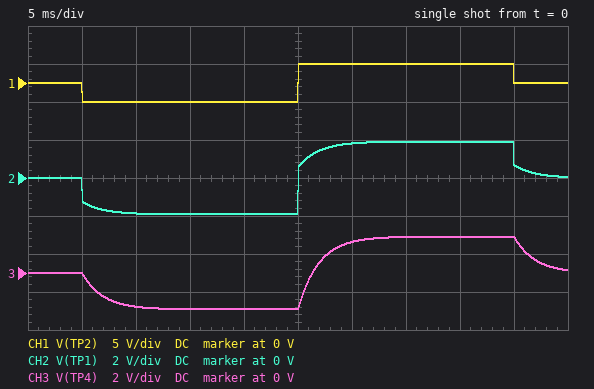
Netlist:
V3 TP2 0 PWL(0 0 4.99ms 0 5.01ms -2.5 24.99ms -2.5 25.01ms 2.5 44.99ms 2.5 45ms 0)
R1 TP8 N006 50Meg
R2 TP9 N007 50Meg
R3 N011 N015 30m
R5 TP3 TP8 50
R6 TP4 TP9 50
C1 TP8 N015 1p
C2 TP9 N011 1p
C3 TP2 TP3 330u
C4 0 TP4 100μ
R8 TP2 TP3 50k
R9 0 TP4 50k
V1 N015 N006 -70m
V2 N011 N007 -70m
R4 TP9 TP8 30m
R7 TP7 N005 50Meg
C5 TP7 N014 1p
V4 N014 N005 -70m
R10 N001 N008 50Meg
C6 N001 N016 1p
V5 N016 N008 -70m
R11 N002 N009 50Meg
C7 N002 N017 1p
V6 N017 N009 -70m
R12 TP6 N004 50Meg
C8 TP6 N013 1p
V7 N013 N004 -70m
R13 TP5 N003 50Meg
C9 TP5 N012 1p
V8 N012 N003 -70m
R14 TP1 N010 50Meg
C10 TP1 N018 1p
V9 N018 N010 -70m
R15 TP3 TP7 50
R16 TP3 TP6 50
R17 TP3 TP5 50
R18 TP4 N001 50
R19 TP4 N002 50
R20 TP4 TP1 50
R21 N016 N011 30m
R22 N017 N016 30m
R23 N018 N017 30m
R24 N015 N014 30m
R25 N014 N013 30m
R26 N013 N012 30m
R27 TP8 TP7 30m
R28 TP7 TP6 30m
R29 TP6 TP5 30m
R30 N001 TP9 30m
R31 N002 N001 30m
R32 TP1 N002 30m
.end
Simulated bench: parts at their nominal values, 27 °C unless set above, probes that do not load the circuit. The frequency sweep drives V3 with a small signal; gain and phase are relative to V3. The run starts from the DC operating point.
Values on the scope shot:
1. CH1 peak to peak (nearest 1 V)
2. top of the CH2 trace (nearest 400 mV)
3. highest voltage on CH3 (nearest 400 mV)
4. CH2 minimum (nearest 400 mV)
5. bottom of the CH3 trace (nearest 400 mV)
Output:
5 V
2.0 V
2.0 V
-2.0 V
-2.0 V
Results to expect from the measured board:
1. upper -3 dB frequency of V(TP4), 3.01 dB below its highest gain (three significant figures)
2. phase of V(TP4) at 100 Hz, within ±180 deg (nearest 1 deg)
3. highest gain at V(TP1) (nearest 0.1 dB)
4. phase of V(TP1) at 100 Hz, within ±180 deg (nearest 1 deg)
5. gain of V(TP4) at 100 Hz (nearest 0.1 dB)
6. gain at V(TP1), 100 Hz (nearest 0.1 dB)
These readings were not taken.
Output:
82.7 Hz
-50 deg
-2.3 dB
-12 deg
-6.2 dB
-4.1 dB
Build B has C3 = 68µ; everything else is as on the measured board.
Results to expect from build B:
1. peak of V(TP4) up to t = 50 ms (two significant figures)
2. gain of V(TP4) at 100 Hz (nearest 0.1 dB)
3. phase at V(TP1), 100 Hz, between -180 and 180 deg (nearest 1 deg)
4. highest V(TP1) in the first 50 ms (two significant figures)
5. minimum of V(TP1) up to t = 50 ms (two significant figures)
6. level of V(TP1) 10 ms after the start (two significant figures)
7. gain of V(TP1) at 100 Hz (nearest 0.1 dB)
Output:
1.0 V
-9.3 dB
6 deg
1.5 V
-1.2 V
-1.0 V
-7.3 dB
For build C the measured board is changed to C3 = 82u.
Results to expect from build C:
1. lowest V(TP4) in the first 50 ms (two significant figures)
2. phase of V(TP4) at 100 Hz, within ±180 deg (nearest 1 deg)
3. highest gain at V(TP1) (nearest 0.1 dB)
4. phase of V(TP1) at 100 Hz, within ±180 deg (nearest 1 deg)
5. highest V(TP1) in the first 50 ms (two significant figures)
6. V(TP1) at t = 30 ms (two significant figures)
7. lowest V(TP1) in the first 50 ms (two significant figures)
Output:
-1.1 V
-35 deg
-6.1 dB
3 deg
1.4 V
1.1 V
-1.2 V
